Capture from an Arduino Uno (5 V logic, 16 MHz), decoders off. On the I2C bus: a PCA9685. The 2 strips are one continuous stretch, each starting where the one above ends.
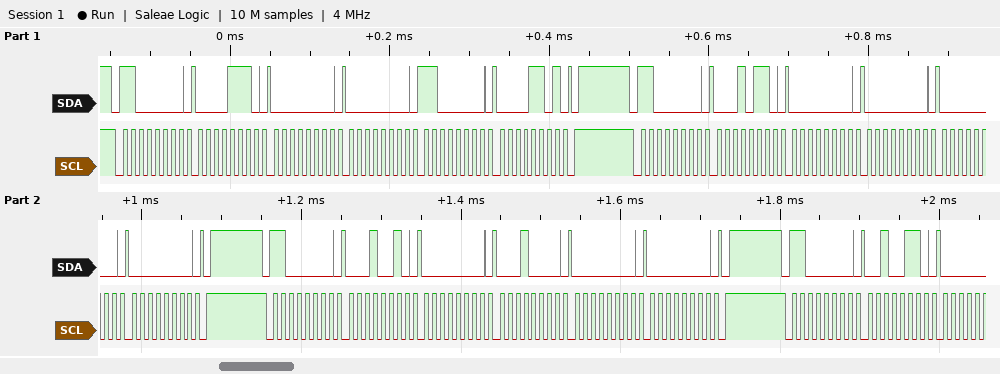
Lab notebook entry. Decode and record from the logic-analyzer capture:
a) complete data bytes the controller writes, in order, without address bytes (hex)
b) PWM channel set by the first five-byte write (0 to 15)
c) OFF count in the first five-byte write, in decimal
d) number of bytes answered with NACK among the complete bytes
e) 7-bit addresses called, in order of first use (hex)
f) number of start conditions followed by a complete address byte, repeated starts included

0E 00 00 C0 0D 16 00 00 00 00 12 00 10 00 00 26
2
3520
0
0x60
4
